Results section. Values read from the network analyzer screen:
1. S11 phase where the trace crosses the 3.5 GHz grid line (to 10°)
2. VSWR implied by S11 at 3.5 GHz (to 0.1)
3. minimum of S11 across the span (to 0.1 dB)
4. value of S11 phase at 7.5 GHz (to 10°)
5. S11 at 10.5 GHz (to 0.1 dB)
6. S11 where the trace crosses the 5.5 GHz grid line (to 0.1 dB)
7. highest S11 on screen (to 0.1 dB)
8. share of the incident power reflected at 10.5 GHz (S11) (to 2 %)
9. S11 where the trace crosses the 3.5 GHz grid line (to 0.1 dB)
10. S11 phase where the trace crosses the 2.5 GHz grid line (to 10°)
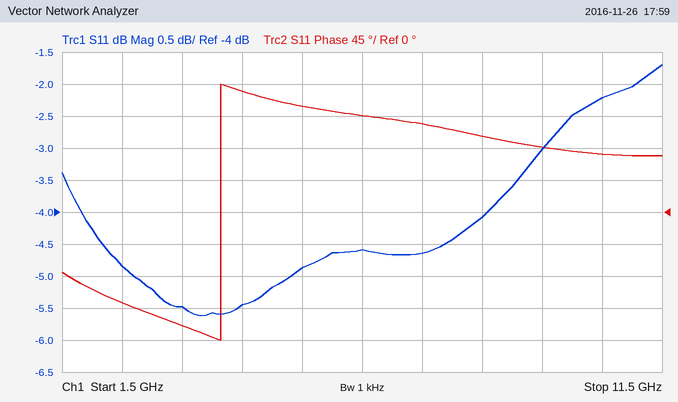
-160°
3.3
-5.6 dB
120°
-2.2 dB
-4.9 dB
-1.7 dB
60 %
-5.5 dB
-130°
